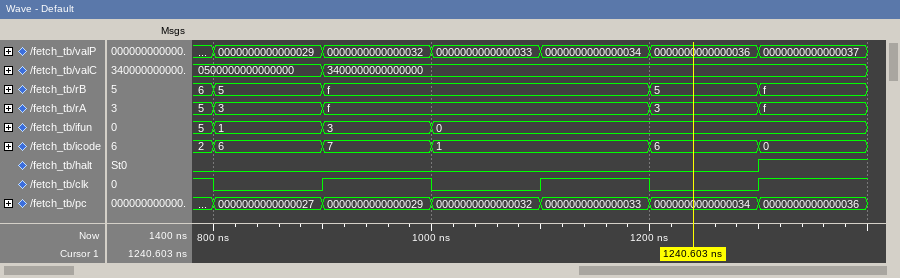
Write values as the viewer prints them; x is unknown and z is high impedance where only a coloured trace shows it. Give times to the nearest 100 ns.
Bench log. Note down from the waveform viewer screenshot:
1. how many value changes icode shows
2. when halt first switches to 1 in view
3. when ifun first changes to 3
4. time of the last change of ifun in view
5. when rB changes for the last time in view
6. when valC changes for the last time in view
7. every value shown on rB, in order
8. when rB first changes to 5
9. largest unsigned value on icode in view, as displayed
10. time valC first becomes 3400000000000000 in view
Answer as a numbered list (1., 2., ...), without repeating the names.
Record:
1. 5
2. 1300 ns
3. 900 ns
4. 1000 ns
5. 1300 ns
6. 900 ns
7. 6, 5, f, 5, f
8. 800 ns
9. 7
10. 900 ns
